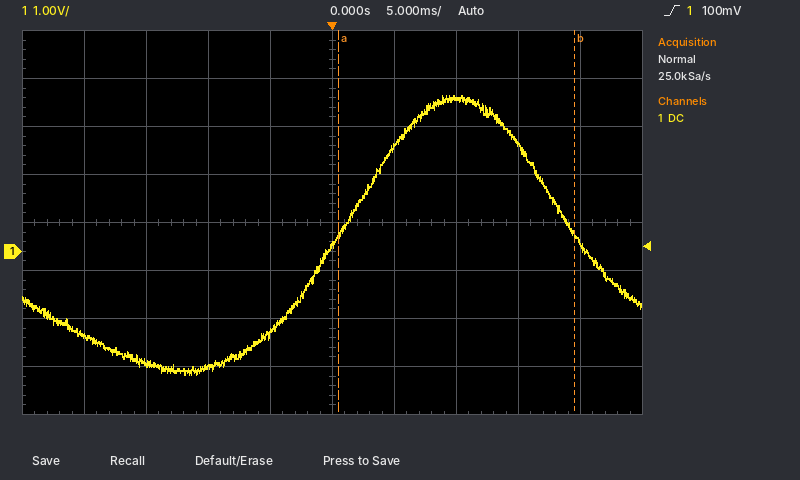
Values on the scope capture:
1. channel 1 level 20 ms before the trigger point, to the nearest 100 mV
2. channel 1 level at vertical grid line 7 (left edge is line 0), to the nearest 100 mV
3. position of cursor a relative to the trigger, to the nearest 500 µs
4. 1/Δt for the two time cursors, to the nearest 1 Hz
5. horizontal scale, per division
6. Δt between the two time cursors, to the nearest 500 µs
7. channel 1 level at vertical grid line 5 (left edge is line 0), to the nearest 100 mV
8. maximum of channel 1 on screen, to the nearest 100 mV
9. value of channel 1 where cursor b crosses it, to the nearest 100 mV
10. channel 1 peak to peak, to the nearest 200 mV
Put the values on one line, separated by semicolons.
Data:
-1.8 V; 3.2 V; +500 µs; 53 Hz; 5 ms; 19.0 ms; 100 mV; 3.2 V; 400 mV; 5.8 V
